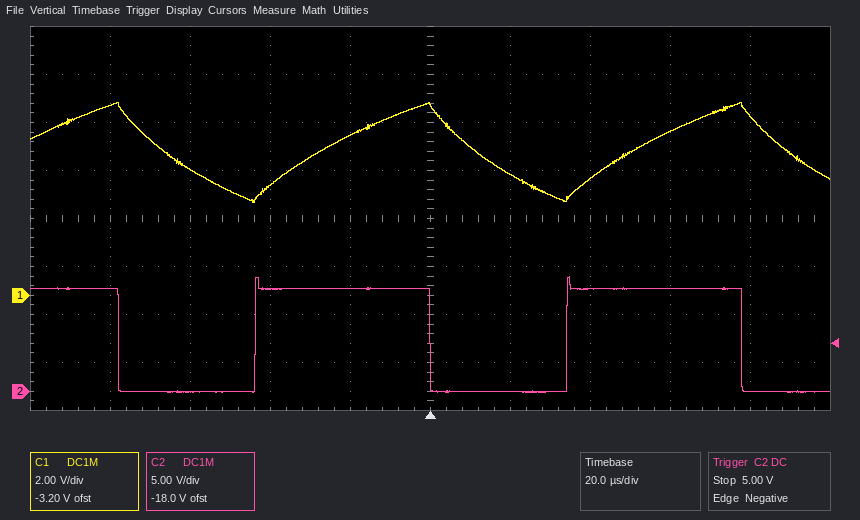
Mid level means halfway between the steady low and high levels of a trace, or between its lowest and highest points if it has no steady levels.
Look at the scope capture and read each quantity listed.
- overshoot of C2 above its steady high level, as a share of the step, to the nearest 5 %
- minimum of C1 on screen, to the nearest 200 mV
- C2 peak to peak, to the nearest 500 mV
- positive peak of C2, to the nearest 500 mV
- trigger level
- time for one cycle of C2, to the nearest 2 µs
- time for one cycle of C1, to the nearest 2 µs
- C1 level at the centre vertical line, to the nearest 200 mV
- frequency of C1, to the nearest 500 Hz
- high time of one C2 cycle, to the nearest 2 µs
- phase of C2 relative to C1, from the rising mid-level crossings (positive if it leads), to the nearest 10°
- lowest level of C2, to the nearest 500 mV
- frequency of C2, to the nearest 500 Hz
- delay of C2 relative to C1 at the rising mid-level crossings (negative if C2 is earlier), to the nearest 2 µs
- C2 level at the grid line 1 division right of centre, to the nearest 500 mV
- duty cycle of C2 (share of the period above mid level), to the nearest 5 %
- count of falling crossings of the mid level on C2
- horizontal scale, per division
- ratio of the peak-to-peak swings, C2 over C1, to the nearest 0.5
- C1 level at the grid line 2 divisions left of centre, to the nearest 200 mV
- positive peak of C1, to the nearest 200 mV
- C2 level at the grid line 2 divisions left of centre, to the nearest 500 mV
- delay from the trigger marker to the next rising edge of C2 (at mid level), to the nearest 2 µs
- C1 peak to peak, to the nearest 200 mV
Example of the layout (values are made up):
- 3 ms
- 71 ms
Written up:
- 10 %
- 3.8 V
- 12.0 V
- 12.0 V
- 5.00 V
- 78 µs
- 78 µs
- 7.8 V
- 13.0 kHz
- 44 µs
- +70°
- 0.0 V
- 13.0 kHz
- -16 µs
- 0.0 V
- 55 %
- 3
- 20 µs
- 3.0
- 4.6 V
- 8.0 V
- 10.5 V
- 34 µs
- 4.2 V
